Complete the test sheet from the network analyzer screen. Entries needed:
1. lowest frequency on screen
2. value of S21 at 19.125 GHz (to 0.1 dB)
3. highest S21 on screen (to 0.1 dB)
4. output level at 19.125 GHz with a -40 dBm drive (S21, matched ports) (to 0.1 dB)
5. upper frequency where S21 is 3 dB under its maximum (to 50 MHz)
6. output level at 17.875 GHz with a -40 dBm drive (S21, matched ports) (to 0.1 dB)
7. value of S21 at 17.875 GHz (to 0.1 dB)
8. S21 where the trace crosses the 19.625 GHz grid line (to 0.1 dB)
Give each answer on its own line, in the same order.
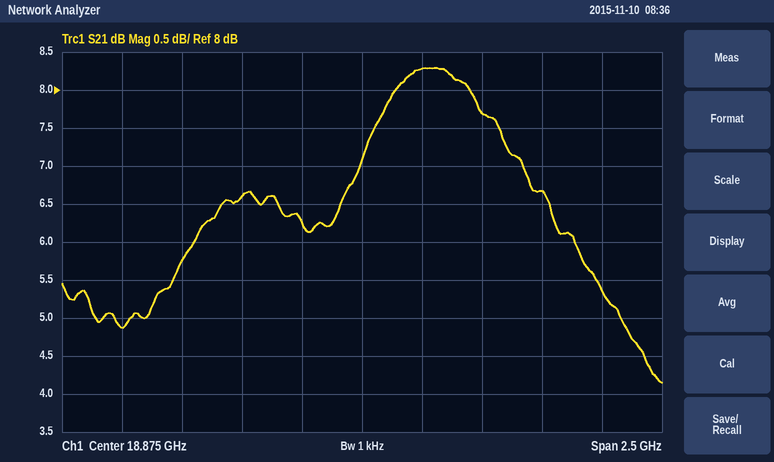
17.625 GHz
8.3 dB
8.3 dB
-31.7 dBm
19.90 GHz
-35.1 dBm
4.9 dB
6.7 dB
